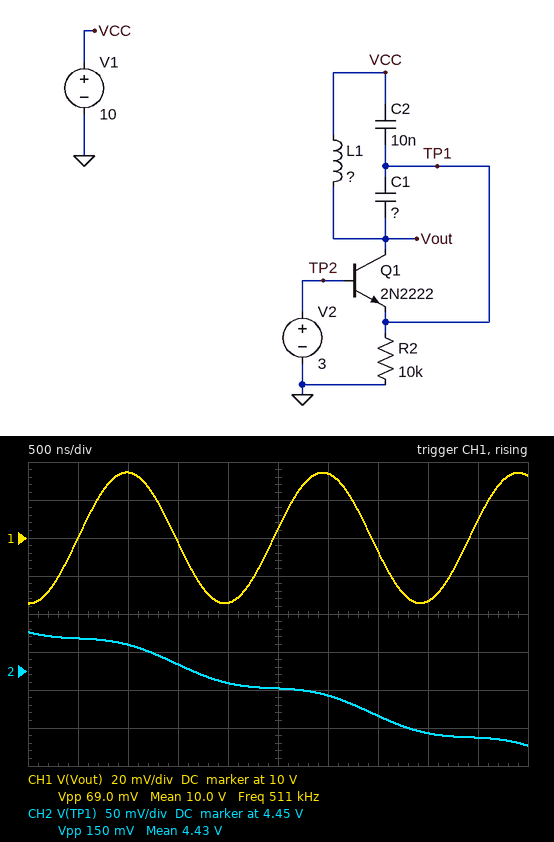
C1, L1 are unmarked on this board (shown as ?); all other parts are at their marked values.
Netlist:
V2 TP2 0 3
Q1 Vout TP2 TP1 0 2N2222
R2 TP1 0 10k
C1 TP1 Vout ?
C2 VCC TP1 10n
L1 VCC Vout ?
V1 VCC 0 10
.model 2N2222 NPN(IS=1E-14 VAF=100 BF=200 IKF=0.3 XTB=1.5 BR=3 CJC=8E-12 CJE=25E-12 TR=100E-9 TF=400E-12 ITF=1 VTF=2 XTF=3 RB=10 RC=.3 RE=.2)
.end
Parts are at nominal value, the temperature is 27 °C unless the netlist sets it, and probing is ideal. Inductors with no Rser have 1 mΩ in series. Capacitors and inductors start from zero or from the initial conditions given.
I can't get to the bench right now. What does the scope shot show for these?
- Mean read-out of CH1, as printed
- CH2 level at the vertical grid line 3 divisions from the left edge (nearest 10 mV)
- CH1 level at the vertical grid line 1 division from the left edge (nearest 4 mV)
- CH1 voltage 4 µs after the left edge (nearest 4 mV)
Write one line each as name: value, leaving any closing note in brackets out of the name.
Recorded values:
Mean read-out of CH1, as printed: 10.0 V
CH2 level at the vertical grid line 3 divisions from the left edge: 4.46 V
CH1 level at the vertical grid line 1 division from the left edge: 10.000 V
CH1 voltage 4 µs after the left edge: 9.968 V
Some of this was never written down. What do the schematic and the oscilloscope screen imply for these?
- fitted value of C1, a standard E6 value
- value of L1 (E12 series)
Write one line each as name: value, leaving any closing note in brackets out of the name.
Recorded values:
fitted value of C1, a standard E6 value: 3.3 nF
value of L1: 39 µH
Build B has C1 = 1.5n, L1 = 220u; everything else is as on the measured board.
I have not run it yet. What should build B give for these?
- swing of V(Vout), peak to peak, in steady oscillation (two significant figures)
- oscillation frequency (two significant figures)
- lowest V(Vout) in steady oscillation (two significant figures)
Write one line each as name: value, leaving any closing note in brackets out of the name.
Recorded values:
swing of V(Vout), peak to peak, in steady oscillation: 120 mV
oscillation frequency: 300 kHz
lowest V(Vout) in steady oscillation: 9.9 V
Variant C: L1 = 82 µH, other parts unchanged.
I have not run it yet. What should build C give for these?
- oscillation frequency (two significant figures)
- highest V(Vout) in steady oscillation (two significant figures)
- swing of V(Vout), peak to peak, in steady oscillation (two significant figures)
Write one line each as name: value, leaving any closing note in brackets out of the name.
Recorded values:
oscillation frequency: 350 kHz
highest V(Vout) in steady oscillation: 10 V
swing of V(Vout), peak to peak, in steady oscillation: 90 mV
